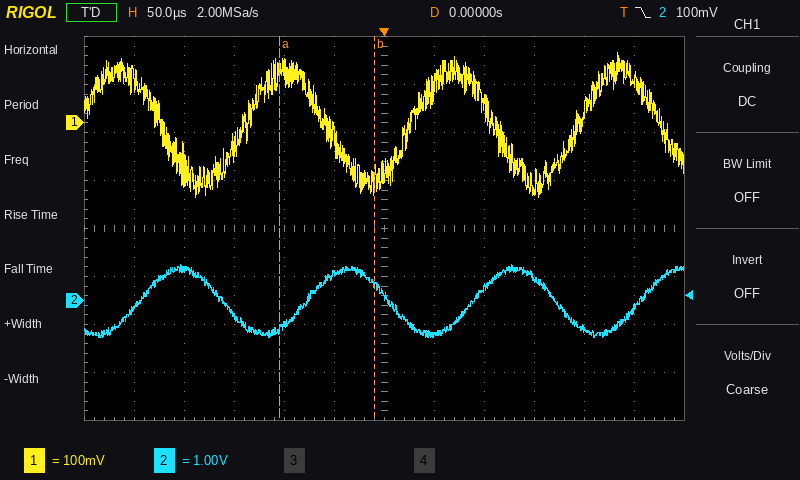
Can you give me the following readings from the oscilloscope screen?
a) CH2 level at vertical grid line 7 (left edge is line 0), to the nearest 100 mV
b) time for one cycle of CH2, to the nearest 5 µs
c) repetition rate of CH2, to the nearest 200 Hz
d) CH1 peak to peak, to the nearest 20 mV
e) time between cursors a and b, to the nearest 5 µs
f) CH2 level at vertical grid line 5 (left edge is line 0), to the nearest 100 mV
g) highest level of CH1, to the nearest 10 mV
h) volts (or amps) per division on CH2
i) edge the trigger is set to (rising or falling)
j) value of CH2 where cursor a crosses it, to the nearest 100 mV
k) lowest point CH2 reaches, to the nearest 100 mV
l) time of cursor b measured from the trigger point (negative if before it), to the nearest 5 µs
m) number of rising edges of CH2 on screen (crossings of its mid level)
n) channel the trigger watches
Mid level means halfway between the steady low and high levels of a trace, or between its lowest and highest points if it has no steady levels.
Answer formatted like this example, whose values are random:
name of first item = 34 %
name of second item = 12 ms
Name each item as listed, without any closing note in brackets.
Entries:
CH2 level at vertical grid line 7 (left edge is line 0), to the nearest 100 mV = -700 mV
time for one cycle of CH2, to the nearest 5 µs = 165 µs
repetition rate of CH2, to the nearest 200 Hz = 6.0 kHz
CH1 peak to peak, to the nearest 20 mV = 300 mV
time between cursors a and b, to the nearest 5 µs = 95 µs
CH2 level at vertical grid line 5 (left edge is line 0), to the nearest 100 mV = 500 mV
highest level of CH1, to the nearest 10 mV = 150 mV
volts (or amps) per division on CH2 = 1 V
edge the trigger is set to = falling
value of CH2 where cursor a crosses it, to the nearest 100 mV = -600 mV
lowest point CH2 reaches, to the nearest 100 mV = -800 mV
time of cursor b measured from the trigger point (negative if before it), to the nearest 5 µs = -10 µs
number of rising edges of CH2 on screen = 4
channel the trigger watches = CH2
